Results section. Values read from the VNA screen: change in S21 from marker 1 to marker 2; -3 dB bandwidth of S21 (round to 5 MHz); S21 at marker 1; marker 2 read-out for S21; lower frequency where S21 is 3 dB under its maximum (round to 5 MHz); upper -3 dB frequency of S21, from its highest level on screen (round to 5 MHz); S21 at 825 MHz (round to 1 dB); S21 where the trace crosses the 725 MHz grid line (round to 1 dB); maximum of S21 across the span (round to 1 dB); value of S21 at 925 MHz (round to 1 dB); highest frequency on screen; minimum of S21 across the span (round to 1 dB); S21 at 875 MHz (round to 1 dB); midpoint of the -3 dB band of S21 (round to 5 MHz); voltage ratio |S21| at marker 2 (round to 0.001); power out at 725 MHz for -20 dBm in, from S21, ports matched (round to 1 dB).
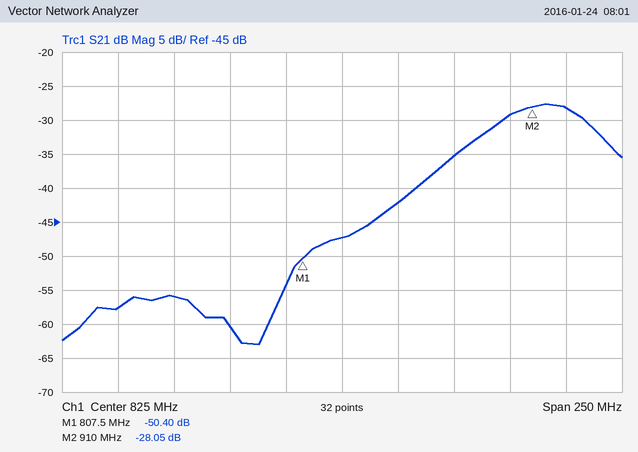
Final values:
22.35 dB
40 MHz
-50.40 dB
-28.05 dB
895 MHz
935 MHz
-47 dB
-58 dB
-28 dB
-28 dB
950 MHz
-63 dB
-35 dB
915 MHz
0.040
-78 dBm
